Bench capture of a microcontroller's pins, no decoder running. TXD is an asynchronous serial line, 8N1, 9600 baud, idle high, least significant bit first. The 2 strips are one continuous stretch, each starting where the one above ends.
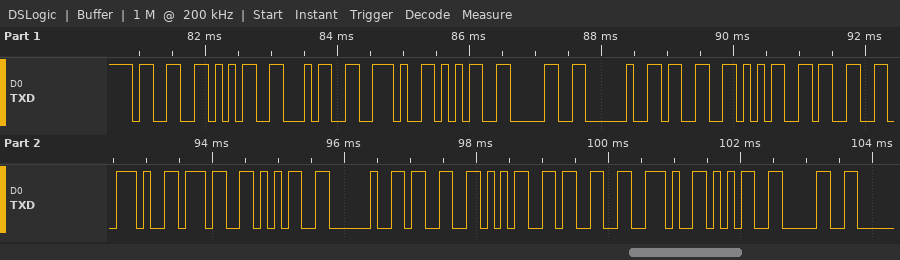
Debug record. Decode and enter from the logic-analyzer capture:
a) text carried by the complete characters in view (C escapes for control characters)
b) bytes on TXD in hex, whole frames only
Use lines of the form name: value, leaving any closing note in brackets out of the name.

text carried by the complete characters in view: "354.50 353.75 353.50"
bytes on TXD in hex, whole frames only: 0x33 0x35 0x34 0x2E 0x35 0x30 0x20 0x33 0x35 0x33 0x2E 0x37 0x35 0x20 0x33 0x35 0x33 0x2E 0x35 0x30
